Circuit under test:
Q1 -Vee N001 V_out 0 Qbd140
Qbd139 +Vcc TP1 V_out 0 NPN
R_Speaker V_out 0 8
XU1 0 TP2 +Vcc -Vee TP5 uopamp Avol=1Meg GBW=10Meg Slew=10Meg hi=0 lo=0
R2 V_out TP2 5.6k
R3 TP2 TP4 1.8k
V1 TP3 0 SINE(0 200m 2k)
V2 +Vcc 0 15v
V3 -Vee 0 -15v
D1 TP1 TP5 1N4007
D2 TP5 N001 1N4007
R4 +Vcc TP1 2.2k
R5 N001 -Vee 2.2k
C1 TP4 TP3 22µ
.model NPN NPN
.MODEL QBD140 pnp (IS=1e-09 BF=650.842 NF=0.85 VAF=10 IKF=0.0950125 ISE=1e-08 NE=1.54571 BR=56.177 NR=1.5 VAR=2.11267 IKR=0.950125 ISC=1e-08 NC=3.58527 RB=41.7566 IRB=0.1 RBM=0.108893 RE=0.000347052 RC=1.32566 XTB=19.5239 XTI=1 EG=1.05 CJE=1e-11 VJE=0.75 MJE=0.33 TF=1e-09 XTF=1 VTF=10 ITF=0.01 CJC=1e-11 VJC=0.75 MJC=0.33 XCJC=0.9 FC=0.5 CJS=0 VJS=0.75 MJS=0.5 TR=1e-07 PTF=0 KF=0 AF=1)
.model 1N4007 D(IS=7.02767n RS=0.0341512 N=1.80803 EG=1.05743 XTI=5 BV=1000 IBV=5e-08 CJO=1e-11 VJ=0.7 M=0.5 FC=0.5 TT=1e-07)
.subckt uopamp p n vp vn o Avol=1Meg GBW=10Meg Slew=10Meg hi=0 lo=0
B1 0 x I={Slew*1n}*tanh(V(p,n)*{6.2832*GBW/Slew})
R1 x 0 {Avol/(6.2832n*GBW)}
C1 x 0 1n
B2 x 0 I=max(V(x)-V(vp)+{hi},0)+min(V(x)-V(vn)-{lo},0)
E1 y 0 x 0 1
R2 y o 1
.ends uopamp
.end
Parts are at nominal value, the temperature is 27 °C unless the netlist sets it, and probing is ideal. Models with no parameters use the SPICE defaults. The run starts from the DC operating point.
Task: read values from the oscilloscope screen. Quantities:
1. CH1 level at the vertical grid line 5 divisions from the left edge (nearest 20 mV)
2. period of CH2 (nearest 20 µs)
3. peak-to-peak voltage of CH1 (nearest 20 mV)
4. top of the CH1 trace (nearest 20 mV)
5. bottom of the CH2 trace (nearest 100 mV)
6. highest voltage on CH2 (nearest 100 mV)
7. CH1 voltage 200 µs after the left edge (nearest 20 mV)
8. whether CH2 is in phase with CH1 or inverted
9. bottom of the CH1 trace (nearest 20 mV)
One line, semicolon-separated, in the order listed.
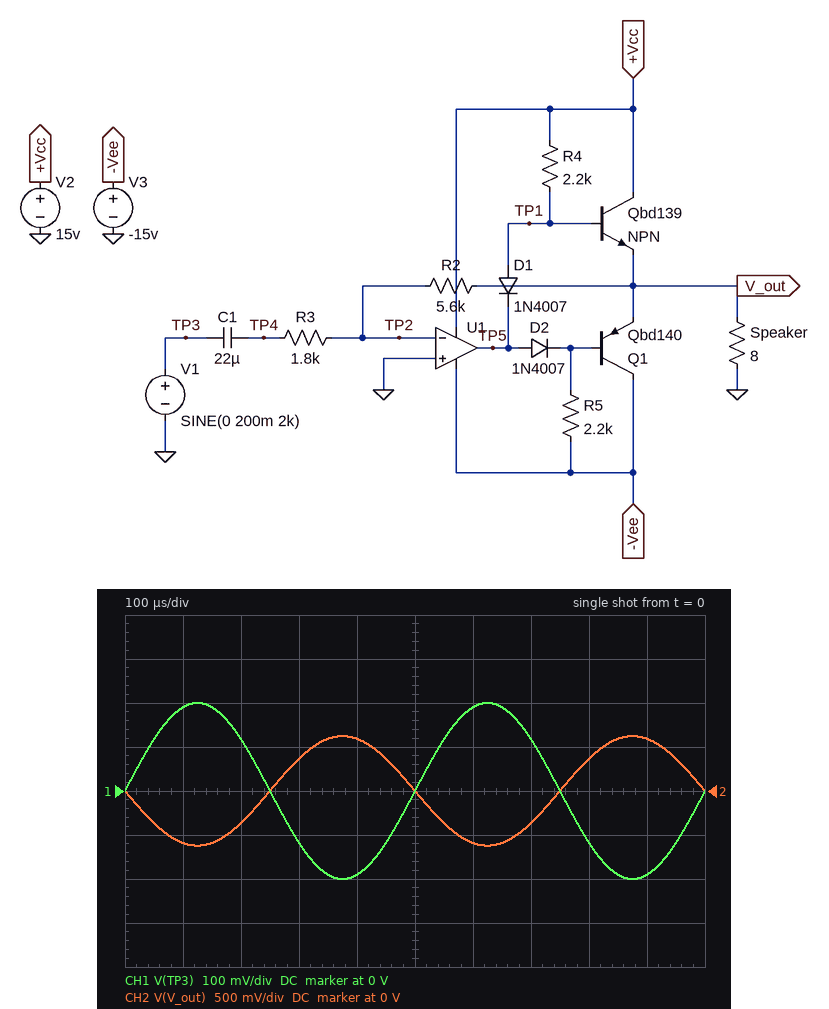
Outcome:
0 V; 500 µs; 400 mV; 200 mV; -600 mV; 600 mV; 120 mV; inverted; -200 mV
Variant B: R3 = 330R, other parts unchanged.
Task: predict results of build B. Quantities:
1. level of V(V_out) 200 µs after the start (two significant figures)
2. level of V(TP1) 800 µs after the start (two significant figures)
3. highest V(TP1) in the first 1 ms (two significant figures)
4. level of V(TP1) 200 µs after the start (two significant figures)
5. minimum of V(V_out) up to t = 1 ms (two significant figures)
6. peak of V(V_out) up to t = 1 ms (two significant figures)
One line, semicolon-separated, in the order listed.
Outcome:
-1.9 V; 3.0 V; 4.4 V; -1.1 V; -3.4 V; 3.4 V
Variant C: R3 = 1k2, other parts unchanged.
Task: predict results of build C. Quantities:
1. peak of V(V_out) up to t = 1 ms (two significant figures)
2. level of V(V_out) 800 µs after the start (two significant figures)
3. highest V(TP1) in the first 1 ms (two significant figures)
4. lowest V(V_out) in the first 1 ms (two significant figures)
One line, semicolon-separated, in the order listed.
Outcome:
940 mV; 550 mV; 1.8 V; -930 mV
